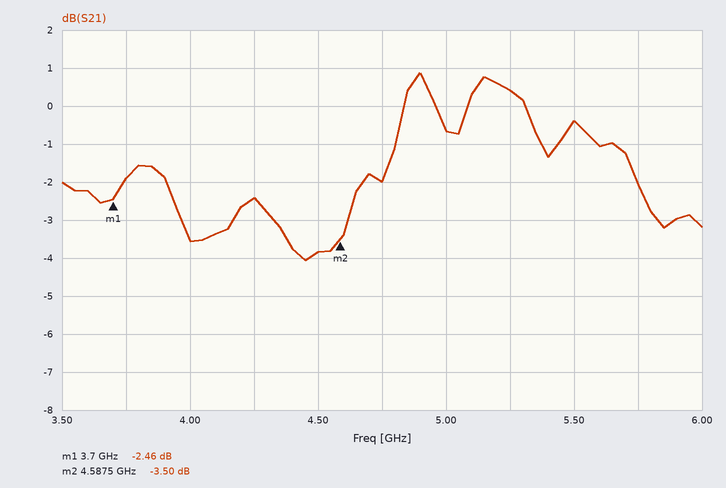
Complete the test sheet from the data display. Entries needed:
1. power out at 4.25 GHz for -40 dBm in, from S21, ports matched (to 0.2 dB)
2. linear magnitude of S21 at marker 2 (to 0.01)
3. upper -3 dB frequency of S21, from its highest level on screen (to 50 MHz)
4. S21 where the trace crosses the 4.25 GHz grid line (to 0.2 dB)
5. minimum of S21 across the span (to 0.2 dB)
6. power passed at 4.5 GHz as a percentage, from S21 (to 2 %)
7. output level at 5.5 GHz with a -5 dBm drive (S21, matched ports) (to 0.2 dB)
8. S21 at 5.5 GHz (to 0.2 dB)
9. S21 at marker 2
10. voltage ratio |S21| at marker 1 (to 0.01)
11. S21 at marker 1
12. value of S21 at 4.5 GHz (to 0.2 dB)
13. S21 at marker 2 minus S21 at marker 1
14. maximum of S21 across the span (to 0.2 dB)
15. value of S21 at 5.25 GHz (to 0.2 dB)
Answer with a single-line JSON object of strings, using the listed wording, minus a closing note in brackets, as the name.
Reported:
{"power out at 4.25 GHz for -40 dBm in, from S21, ports matched": "-42.4 dBm", "linear magnitude of S21 at marker 2": "0.67", "upper -3 dB frequency of S21, from its highest level on screen": "5.75 GHz", "S21 where the trace crosses the 4.25 GHz grid line": "-2.4 dB", "minimum of S21 across the span": "-4.0 dB", "power passed at 4.5 GHz as a percentage, from S21": "42 %", "output level at 5.5 GHz with a -5 dBm drive (S21, matched ports)": "-5.4 dBm", "S21 at 5.5 GHz": "-0.4 dB", "S21 at marker 2": "-3.50 dB", "voltage ratio |S21| at marker 1": "0.75", "S21 at marker 1": "-2.46 dB", "value of S21 at 4.5 GHz": "-3.8 dB", "S21 at marker 2 minus S21 at marker 1": "-1.04 dB", "maximum of S21 across the span": "0.8 dB", "value of S21 at 5.25 GHz": "0.4 dB"}
